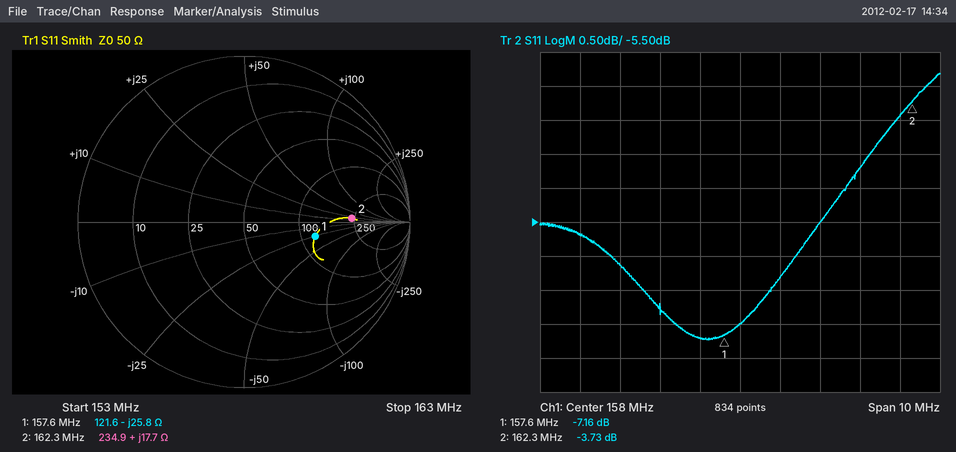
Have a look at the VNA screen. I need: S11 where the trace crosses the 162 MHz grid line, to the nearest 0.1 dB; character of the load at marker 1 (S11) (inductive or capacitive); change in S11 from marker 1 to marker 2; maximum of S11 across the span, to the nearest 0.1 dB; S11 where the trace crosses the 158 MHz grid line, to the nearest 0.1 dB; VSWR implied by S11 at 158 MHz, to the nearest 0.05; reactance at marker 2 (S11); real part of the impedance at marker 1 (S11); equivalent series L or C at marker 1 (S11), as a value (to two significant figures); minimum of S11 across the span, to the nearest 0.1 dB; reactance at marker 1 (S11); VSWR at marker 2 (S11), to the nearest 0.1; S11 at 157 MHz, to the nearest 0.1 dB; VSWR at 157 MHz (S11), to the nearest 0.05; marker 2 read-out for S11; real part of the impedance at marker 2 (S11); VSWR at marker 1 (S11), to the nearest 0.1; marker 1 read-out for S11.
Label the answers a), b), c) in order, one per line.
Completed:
a) -3.9 dB
b) capacitive
c) 3.43 dB
d) -3.3 dB
e) -7.0 dB
f) 2.60
g) +17.7 Ω
h) 121.6 Ω
i) 39 pF
j) -7.2 dB
k) -25.8 Ω
l) 4.7
m) -7.2 dB
n) 2.55
o) -3.73 dB
p) 234.9 Ω
q) 2.6
r) -7.16 dB
